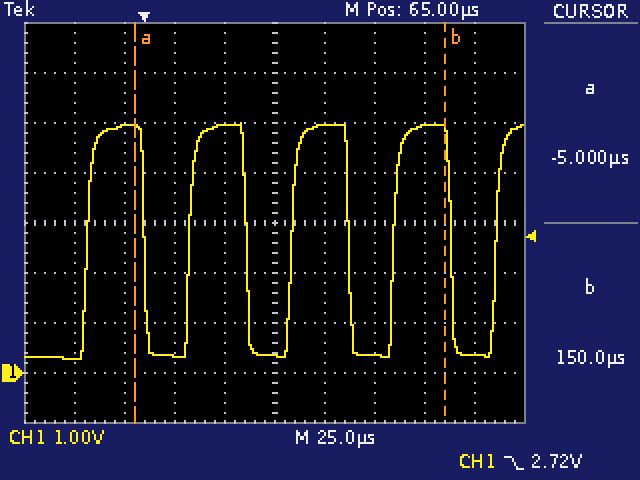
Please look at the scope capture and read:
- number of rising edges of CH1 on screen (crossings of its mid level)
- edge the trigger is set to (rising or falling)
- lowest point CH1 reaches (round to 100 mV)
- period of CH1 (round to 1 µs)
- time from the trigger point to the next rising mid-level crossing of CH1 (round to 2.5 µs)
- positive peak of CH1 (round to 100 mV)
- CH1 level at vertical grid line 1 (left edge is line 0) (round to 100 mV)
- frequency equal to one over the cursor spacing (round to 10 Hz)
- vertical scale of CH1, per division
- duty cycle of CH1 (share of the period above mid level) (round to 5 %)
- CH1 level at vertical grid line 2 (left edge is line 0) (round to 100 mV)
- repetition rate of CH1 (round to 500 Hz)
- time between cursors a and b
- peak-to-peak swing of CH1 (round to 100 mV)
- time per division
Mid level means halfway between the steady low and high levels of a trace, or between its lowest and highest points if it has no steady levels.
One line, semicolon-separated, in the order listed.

5; falling; 300 mV; 51 µs; 22.5 µs; 5.0 V; 300 mV; 6.45 kHz; 1 V; 55 %; 4.9 V; 19.5 kHz; 155.0 µs; 4.7 V; 25 µs
